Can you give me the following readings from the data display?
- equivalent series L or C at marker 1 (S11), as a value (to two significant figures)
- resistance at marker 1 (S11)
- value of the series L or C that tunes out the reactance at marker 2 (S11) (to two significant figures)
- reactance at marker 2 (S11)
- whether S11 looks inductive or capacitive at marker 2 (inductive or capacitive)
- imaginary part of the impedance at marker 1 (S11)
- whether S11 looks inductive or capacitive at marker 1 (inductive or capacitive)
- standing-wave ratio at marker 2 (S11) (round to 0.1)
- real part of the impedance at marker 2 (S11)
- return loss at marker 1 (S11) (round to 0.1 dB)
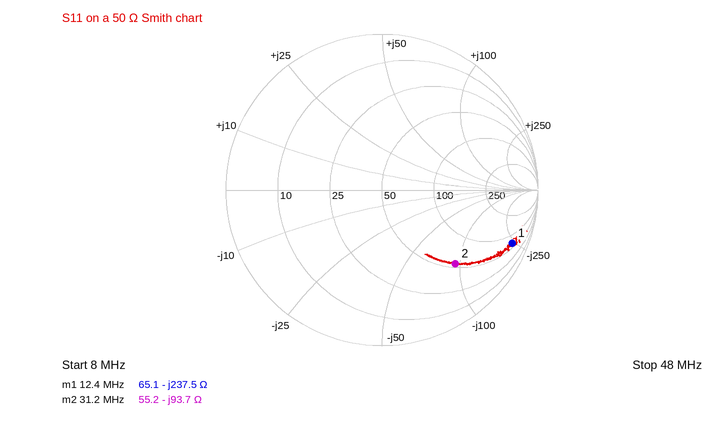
54 pF
65.1 Ω
480 nH
-93.7 Ω
capacitive
-237.5 Ω
capacitive
5.0
55.2 Ω
0.9 dB
